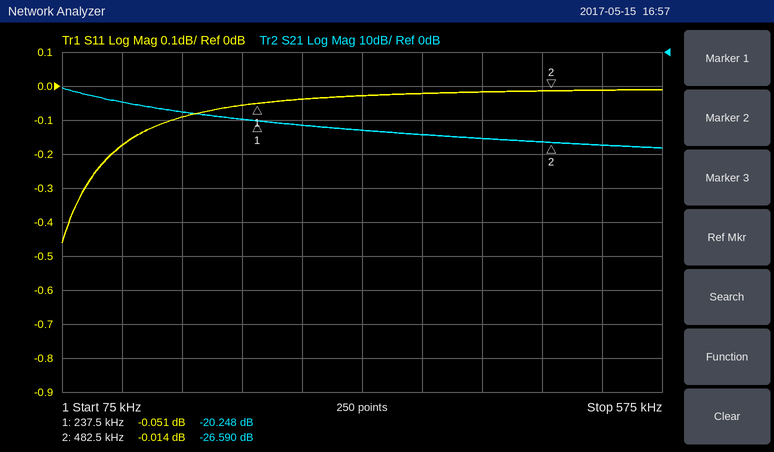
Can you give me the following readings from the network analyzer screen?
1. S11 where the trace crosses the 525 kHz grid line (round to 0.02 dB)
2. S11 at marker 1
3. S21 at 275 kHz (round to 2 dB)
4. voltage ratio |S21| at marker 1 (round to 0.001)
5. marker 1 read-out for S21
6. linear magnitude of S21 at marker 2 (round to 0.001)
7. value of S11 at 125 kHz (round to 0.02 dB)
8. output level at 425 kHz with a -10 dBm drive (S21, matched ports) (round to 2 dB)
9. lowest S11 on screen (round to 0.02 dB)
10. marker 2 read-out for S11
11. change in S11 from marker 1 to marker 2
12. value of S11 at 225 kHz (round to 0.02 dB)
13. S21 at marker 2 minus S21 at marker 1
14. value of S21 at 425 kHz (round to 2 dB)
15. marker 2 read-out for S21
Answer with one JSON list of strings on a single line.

["-0.02 dB", "-0.051 dB", "-22 dB", "0.097", "-20.248 dB", "0.047", "-0.18 dB", "-36 dBm", "-0.46 dB", "-0.014 dB", "0.037 dB", "-0.06 dB", "-6.342 dB", "-26 dB", "-26.590 dB"]
